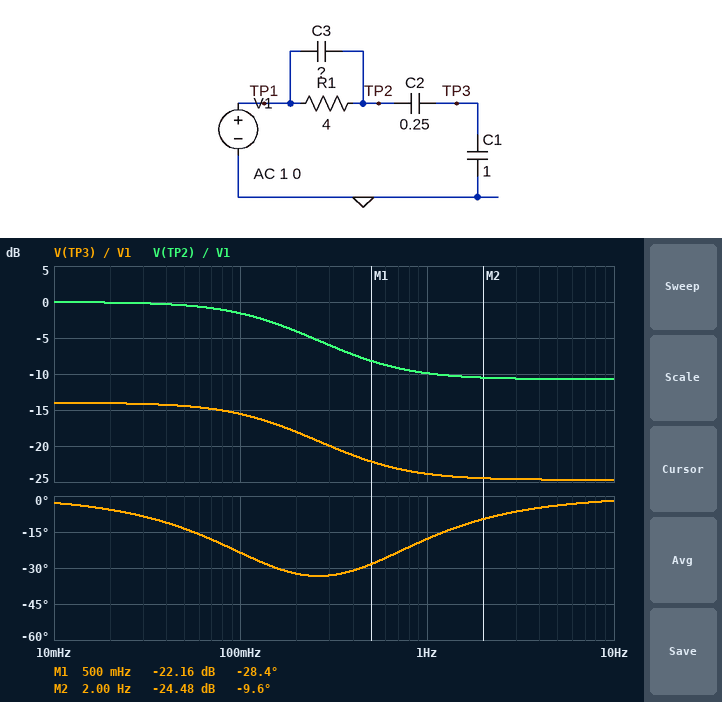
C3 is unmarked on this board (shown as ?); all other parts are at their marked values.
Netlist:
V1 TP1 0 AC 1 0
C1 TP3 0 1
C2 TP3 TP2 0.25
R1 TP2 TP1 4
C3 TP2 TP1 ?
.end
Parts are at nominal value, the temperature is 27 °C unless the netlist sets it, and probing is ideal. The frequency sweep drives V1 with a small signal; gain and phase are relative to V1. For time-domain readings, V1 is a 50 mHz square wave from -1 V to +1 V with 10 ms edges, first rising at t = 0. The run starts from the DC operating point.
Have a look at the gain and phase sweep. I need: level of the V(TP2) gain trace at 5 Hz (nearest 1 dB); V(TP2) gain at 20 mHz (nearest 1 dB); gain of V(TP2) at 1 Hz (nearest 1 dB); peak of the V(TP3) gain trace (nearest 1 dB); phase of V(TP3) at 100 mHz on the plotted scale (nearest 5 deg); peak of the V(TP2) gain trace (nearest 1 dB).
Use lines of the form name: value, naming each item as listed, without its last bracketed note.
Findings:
level of the V(TP2) gain trace at 5 Hz: -11 dB
V(TP2) gain at 20 mHz: 0 dB
gain of V(TP2) at 1 Hz: -10 dB
peak of the V(TP3) gain trace: -14 dB
phase of V(TP3) at 100 mHz on the plotted scale: -25 deg
peak of the V(TP2) gain trace: 0 dB
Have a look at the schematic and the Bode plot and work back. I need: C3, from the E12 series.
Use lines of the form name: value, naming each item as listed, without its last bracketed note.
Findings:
C3, from the E12 series: 82 mF
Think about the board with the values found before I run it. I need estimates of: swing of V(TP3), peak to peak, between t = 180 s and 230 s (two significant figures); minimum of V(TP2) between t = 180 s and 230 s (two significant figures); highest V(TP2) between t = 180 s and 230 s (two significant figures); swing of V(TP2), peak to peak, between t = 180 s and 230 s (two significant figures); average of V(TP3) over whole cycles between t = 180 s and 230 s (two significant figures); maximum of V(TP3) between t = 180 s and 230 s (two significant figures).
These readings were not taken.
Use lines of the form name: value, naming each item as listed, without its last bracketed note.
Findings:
swing of V(TP3), peak to peak, between t = 180 s and 230 s: 400 mV
minimum of V(TP2) between t = 180 s and 230 s: -1.0 V
highest V(TP2) between t = 180 s and 230 s: 1.0 V
swing of V(TP2), peak to peak, between t = 180 s and 230 s: 2.0 V
average of V(TP3) over whole cycles between t = 180 s and 230 s: 200 mV
maximum of V(TP3) between t = 180 s and 230 s: 400 mV
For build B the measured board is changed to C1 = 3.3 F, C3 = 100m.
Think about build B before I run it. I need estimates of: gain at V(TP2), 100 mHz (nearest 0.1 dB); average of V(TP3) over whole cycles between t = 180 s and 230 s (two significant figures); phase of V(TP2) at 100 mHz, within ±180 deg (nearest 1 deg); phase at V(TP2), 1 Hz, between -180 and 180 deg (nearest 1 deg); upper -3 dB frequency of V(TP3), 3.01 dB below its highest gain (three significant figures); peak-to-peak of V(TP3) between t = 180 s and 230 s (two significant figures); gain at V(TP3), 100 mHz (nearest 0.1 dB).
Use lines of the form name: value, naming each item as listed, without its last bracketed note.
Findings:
gain at V(TP2), 100 mHz: -2.0 dB
average of V(TP3) over whole cycles between t = 180 s and 230 s: 70 mV
phase of V(TP2) at 100 mHz, within ±180 deg: -26 deg
phase at V(TP2), 1 Hz, between -180 and 180 deg: -15 deg
upper -3 dB frequency of V(TP3), 3.01 dB below its highest gain: 132 mHz
peak-to-peak of V(TP3) between t = 180 s and 230 s: 140 mV
gain at V(TP3), 100 mHz: -25.1 dB
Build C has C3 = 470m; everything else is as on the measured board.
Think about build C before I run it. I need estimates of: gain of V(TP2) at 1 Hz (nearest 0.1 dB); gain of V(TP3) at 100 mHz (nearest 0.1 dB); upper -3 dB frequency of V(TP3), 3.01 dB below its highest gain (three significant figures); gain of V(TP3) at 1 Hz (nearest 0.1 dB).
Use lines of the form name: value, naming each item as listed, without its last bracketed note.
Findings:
gain of V(TP2) at 1 Hz: -3.1 dB
gain of V(TP3) at 100 mHz: -16.0 dB
upper -3 dB frequency of V(TP3), 3.01 dB below its highest gain: 472 mHz
gain of V(TP3) at 1 Hz: -17.0 dB
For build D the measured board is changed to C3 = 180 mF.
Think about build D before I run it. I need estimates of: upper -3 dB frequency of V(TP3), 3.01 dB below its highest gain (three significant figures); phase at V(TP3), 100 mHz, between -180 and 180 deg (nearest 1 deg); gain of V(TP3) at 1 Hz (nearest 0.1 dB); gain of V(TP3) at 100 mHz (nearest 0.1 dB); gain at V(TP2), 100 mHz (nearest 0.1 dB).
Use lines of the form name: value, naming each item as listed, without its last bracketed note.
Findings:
upper -3 dB frequency of V(TP3), 3.01 dB below its highest gain: 141 mHz
phase at V(TP3), 100 mHz, between -180 and 180 deg: -19 deg
gain of V(TP3) at 1 Hz: -20.3 dB
gain of V(TP3) at 100 mHz: -16.0 dB
gain at V(TP2), 100 mHz: -2.0 dB
